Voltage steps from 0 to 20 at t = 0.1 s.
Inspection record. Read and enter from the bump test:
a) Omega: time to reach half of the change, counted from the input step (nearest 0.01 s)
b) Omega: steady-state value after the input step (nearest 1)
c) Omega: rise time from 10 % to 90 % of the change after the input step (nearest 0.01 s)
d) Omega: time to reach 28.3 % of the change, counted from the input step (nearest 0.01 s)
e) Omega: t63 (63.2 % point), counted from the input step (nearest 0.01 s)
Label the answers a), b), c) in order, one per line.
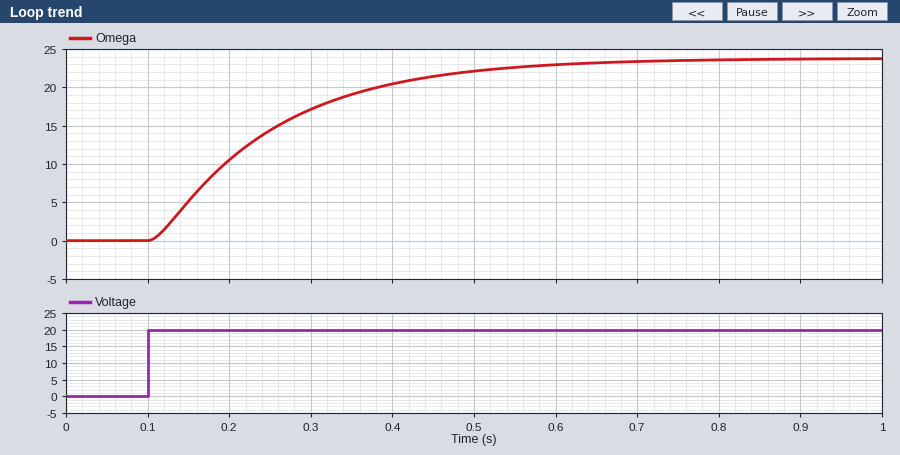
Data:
a) 0.12 s
b) 24
c) 0.32 s
d) 0.06 s
e) 0.16 s
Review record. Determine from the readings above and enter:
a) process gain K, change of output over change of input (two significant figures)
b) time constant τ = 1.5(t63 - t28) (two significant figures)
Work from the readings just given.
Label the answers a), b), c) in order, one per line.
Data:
a) 1.2
b) 0.15 s
